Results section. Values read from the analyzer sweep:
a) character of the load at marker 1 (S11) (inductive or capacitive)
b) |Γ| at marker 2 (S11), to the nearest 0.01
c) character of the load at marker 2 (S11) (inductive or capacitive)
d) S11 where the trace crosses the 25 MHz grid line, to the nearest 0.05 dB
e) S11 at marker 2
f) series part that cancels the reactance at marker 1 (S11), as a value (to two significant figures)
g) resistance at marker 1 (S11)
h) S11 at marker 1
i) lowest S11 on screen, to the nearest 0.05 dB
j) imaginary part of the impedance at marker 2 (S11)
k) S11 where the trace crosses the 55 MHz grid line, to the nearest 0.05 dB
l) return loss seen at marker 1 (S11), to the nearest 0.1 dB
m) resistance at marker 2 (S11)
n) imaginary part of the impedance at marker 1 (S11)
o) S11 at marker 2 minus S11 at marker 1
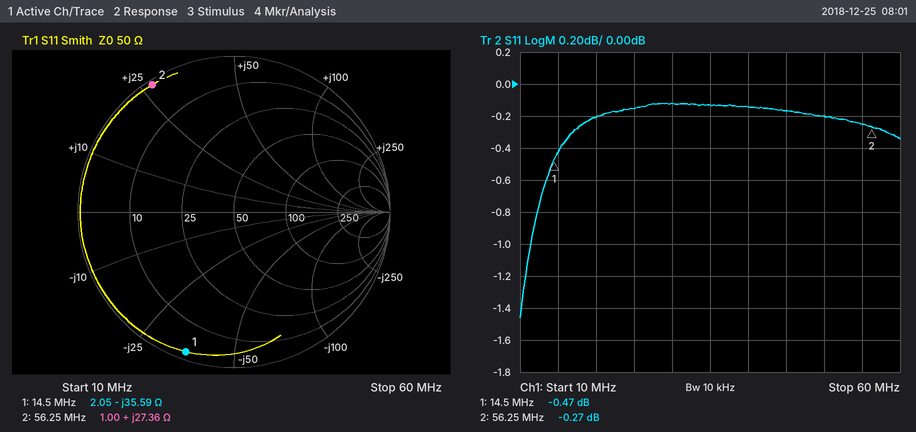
capacitive
0.97
inductive
-0.15 dB
-0.27 dB
390 nH
2.05 Ω
-0.47 dB
-1.45 dB
+27.36 Ω
-0.25 dB
0.5 dB
1.00 Ω
-35.59 Ω
0.20 dB
